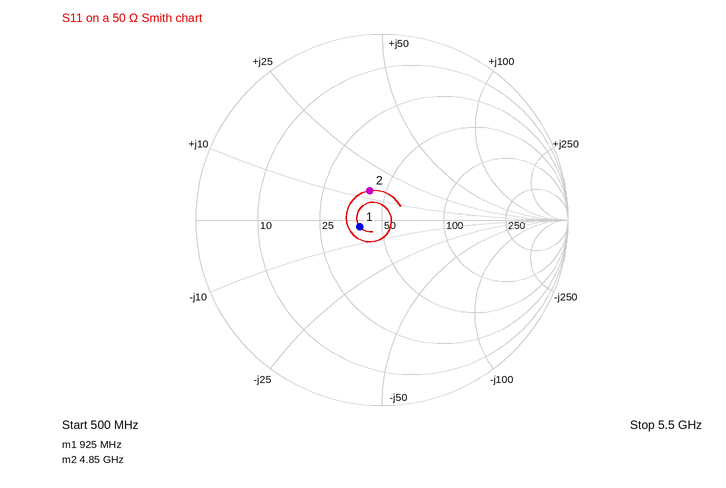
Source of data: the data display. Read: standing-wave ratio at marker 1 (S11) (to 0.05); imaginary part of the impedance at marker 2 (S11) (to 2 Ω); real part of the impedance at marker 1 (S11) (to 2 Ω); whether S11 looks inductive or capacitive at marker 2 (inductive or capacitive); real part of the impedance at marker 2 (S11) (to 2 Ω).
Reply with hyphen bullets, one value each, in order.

- 1.30
- +14 Ω
- 40 Ω
- inductive
- 42 Ω
